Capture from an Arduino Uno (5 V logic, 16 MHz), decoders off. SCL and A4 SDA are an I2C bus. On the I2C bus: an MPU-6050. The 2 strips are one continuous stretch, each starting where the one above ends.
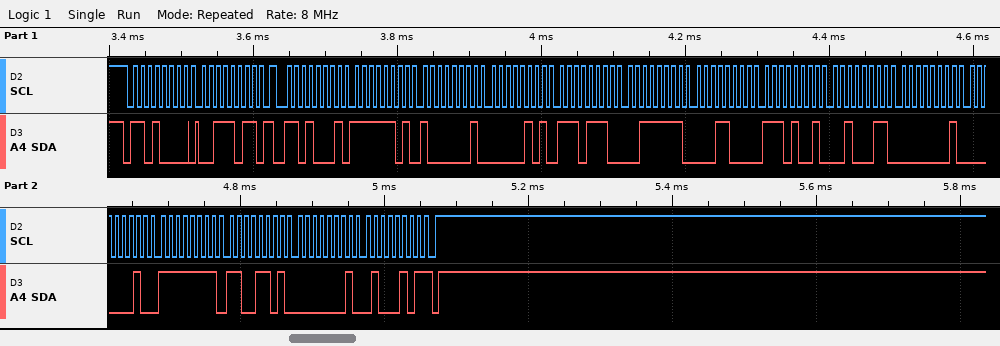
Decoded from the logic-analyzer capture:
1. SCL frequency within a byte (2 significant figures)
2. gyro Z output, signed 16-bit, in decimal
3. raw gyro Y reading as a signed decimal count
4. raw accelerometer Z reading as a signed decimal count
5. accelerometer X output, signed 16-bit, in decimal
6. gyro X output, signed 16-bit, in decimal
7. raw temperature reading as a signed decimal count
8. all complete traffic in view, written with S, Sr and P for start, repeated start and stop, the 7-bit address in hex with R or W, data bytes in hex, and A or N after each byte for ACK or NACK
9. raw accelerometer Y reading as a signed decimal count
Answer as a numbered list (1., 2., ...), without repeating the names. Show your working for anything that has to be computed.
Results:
1. 100 kHz
2. 0x0145 = 325
3. 0xFFCD = -51
4. 0x3F18 = 16152
5. 0xFD81 = -639
6. 0x0102 = 258
7. 0xE923 = -5853
8. S 68W A 3B A Sr 68R A FD A 81 A 05 A EE A 3F A 18 A E9 A 23 A 01 A 02 A FF A CD A 01 A 45 N P
9. 0x05EE = 1518
